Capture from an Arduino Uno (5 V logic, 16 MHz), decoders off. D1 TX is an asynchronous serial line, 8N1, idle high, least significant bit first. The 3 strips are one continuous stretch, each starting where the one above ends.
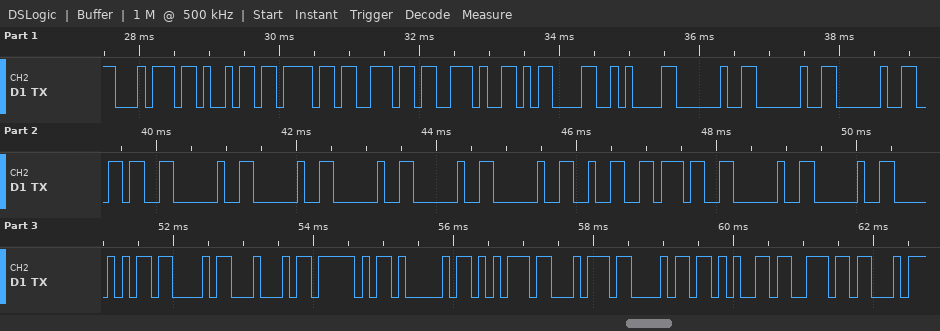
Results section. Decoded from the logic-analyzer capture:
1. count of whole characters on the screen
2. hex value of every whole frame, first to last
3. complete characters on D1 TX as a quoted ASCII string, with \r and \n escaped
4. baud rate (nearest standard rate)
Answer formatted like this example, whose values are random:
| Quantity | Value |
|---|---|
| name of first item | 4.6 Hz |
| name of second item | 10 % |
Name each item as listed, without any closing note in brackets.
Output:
| Quantity | Value |
|---|---|
| count of whole characters on the screen | 30 |
| hex value of every whole frame, first to last | 74 69 6F 6E 2E 0D 0A 20 20 20 36 20 20 20 20 20 32 37 20 20 50 43 44 5F 41 75 74 68 65 6E |
| complete characters on D1 TX as a quoted ASCII string, with \r and \n escaped | "tion.\r\n   6     27  PCD_Authen" |
| baud rate | 9600 baud |
